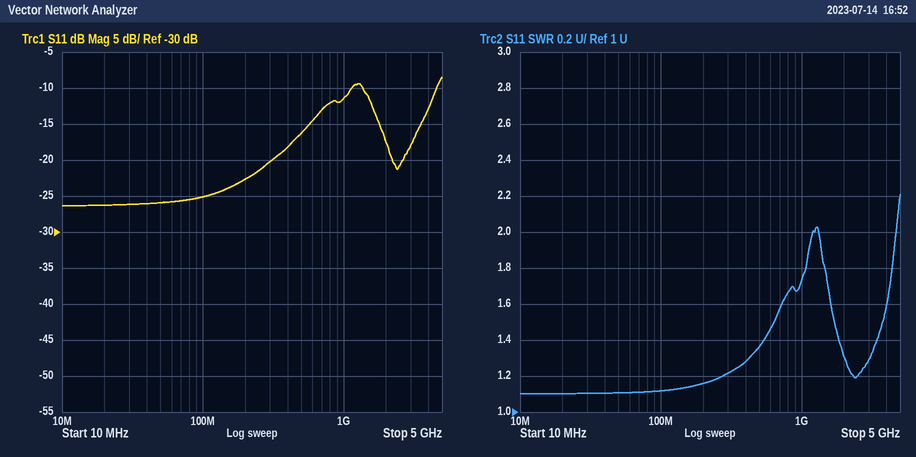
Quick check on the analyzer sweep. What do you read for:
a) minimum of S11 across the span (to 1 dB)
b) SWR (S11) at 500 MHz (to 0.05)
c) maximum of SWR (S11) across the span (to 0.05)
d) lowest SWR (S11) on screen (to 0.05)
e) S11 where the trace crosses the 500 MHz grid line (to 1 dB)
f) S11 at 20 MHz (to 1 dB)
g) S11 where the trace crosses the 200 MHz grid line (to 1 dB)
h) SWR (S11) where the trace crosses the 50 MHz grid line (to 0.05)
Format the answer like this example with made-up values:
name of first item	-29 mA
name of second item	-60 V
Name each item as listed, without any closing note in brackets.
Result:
minimum of S11 across the span	-26 dB
SWR (S11) at 500 MHz	1.35
maximum of SWR (S11) across the span	2.20
lowest SWR (S11) on screen	1.10
S11 where the trace crosses the 500 MHz grid line	-16 dB
S11 at 20 MHz	-26 dB
S11 where the trace crosses the 200 MHz grid line	-23 dB
SWR (S11) where the trace crosses the 50 MHz grid line	1.10
